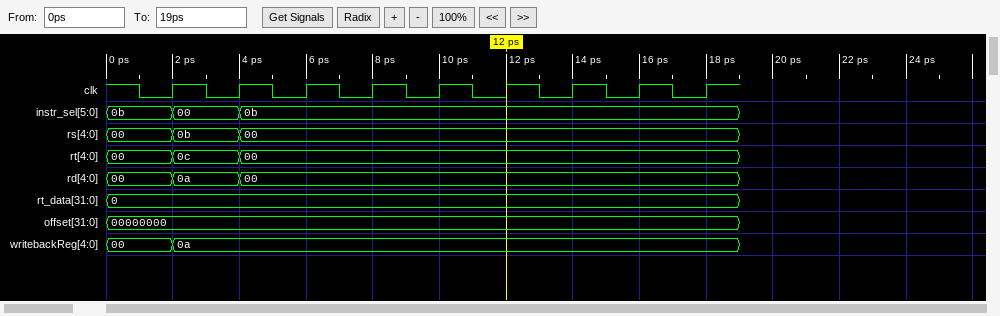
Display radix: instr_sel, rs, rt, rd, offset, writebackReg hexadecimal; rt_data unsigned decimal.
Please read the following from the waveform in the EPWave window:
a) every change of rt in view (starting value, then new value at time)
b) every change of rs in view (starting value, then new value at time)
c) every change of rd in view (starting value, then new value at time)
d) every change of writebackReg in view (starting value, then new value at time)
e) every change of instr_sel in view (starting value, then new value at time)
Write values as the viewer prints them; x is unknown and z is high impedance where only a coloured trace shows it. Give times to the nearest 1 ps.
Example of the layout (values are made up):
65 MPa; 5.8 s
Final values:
00, 0c at 2 ps, 00 at 4 ps; 00, 0b at 2 ps, 00 at 4 ps; 00, 0a at 2 ps, 00 at 4 ps; 00, 0a at 2 ps; 0b, 00 at 2 ps, 0b at 4 ps
